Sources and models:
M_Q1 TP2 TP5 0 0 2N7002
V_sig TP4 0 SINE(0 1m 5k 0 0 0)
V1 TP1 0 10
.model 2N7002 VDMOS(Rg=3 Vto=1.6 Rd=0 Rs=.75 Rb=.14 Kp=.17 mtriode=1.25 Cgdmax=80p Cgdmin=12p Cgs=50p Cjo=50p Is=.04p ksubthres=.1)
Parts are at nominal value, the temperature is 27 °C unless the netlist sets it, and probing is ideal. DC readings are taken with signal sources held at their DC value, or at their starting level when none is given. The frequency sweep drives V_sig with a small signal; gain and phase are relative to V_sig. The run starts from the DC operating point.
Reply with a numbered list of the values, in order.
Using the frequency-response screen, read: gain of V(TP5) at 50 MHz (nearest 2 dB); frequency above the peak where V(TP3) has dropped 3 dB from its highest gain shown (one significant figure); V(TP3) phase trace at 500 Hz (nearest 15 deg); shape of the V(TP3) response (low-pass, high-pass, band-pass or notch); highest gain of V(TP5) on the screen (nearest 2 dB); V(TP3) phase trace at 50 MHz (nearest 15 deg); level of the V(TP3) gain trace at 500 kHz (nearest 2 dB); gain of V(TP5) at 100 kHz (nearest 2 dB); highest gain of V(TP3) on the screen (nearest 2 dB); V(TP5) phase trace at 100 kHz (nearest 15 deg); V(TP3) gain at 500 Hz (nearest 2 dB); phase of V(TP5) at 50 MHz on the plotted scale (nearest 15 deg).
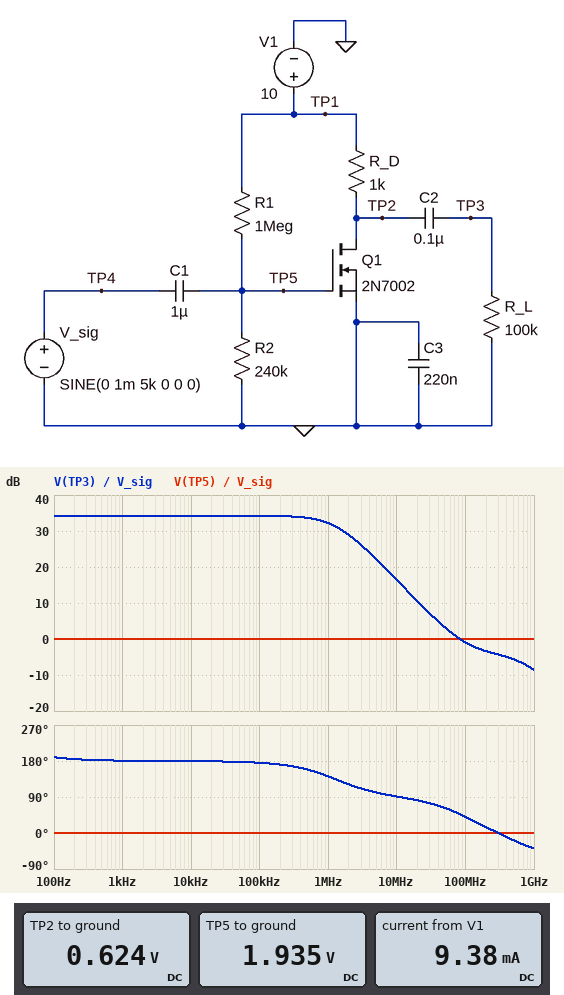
1. 0 dB
2. 1 MHz
3. 180 deg
4. low-pass
5. 0 dB
6. 60 deg
7. 34 dB
8. 0 dB
9. 34 dB
10. 0 deg
11. 34 dB
12. 0 deg
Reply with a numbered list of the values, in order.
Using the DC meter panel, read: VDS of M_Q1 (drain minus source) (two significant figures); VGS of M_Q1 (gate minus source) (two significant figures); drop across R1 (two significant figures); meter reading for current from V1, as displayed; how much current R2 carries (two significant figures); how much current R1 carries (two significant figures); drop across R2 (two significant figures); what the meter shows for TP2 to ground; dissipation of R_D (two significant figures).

1. 620 mV
2. 1.9 V
3. 8.1 V
4. 9.38 mA
5. 8.1 µA
6. 8.1 µA
7. 1.9 V
8. 0.624 V
9. 88 mW
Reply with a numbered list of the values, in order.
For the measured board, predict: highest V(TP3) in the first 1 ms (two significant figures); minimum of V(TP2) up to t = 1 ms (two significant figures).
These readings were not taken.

1. 52 mV
2. 570 mV
